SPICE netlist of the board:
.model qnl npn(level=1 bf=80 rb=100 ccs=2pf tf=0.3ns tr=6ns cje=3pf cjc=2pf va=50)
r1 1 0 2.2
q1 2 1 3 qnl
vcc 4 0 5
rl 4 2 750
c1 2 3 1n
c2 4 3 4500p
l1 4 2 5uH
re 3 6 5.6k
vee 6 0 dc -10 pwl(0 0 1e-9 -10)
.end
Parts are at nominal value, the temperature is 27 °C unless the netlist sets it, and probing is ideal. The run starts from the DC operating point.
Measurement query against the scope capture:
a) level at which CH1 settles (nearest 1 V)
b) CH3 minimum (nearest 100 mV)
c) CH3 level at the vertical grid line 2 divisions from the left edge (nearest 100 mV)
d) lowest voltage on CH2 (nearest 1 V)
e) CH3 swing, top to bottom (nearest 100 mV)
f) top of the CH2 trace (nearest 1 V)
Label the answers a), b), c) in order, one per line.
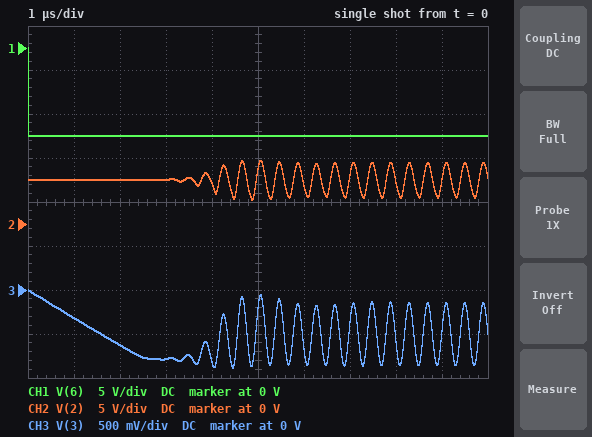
a) -10 V
b) -900 mV
c) -600 mV
d) 3 V
e) 900 mV
f) 7 V
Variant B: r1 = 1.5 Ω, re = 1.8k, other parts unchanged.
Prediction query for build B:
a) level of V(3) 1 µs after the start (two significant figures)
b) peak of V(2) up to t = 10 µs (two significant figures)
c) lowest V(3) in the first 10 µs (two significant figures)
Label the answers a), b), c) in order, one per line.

a) -760 mV
b) 11 V
c) -1.1 V
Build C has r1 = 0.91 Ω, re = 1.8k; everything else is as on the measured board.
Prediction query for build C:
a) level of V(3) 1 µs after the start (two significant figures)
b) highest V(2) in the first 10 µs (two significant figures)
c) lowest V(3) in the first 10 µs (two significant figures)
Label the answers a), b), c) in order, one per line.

a) -760 mV
b) 11 V
c) -1.1 V
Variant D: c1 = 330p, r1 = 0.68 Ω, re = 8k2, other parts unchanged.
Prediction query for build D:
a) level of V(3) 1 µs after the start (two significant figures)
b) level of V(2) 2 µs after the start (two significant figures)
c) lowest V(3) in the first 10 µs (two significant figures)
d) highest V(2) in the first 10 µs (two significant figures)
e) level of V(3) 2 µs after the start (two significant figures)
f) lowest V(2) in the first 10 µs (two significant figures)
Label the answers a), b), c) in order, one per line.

a) -250 mV
b) 5.0 V
c) -820 mV
d) 6.3 V
e) -490 mV
f) 3.7 V
